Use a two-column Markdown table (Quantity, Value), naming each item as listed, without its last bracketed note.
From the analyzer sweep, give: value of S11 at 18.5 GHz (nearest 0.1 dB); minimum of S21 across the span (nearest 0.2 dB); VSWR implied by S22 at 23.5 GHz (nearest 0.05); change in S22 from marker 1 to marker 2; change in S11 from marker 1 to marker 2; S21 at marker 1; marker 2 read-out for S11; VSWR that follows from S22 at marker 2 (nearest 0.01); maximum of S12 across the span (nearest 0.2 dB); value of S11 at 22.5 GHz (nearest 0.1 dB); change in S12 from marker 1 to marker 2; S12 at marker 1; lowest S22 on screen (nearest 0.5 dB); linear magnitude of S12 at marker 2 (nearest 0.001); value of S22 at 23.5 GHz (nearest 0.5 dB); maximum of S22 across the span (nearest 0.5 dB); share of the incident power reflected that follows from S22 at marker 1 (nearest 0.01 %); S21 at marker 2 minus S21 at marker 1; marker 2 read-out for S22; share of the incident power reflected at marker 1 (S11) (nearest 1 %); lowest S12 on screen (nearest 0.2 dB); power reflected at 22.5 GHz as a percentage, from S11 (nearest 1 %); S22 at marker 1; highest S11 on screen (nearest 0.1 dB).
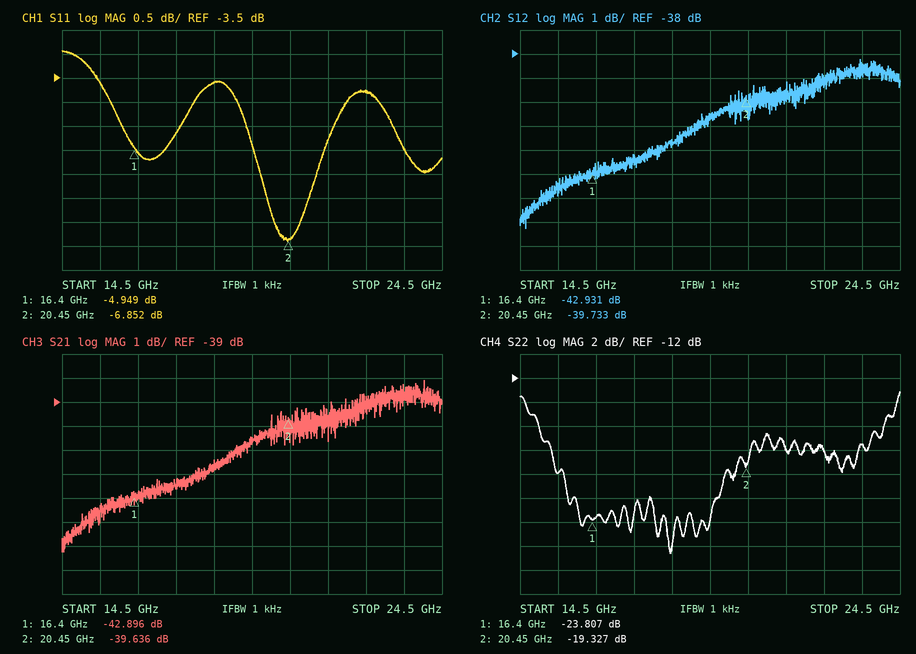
| Quantity | Value |
|---|---|
| value of S11 at 18.5 GHz | -3.6 dB |
| minimum of S21 across the span | -45.2 dB |
| VSWR implied by S22 at 23.5 GHz | 1.30 |
| change in S22 from marker 1 to marker 2 | 4.480 dB |
| change in S11 from marker 1 to marker 2 | -1.903 dB |
| S21 at marker 1 | -42.896 dB |
| marker 2 read-out for S11 | -6.852 dB |
| VSWR that follows from S22 at marker 2 | 1.24 |
| maximum of S12 across the span | -38.2 dB |
| value of S11 at 22.5 GHz | -3.8 dB |
| change in S12 from marker 1 to marker 2 | 3.198 dB |
| S12 at marker 1 | -42.931 dB |
| lowest S22 on screen | -26.5 dB |
| linear magnitude of S12 at marker 2 | 0.010 |
| value of S22 at 23.5 GHz | -17.5 dB |
| maximum of S22 across the span | -13.0 dB |
| share of the incident power reflected that follows from S22 at marker 1 | 0.42 % |
| S21 at marker 2 minus S21 at marker 1 | 3.260 dB |
| marker 2 read-out for S22 | -19.327 dB |
| share of the incident power reflected at marker 1 (S11) | 32 % |
| lowest S12 on screen | -45.2 dB |
| power reflected at 22.5 GHz as a percentage, from S11 | 42 % |
| S22 at marker 1 | -23.807 dB |
| highest S11 on screen | -2.9 dB |
